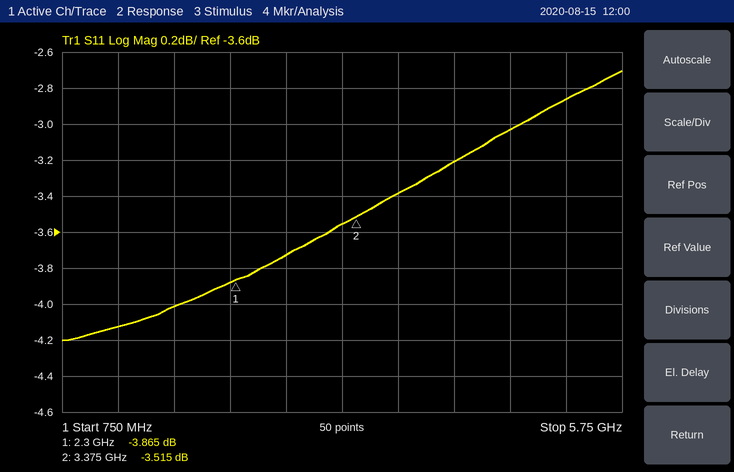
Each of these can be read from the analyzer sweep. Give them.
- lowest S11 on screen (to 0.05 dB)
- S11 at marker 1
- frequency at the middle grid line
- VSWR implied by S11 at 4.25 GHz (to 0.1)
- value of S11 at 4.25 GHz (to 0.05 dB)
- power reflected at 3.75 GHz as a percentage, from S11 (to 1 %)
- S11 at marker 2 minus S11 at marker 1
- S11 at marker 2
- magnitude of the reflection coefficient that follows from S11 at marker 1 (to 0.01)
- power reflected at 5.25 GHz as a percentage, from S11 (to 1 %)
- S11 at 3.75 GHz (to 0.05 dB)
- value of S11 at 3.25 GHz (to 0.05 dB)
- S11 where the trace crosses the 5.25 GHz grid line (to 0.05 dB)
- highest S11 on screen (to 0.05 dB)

-4.20 dB
-3.865 dB
3.25 GHz
5.5
-3.20 dB
46 %
0.350 dB
-3.515 dB
0.64
52 %
-3.40 dB
-3.55 dB
-2.85 dB
-2.70 dB
